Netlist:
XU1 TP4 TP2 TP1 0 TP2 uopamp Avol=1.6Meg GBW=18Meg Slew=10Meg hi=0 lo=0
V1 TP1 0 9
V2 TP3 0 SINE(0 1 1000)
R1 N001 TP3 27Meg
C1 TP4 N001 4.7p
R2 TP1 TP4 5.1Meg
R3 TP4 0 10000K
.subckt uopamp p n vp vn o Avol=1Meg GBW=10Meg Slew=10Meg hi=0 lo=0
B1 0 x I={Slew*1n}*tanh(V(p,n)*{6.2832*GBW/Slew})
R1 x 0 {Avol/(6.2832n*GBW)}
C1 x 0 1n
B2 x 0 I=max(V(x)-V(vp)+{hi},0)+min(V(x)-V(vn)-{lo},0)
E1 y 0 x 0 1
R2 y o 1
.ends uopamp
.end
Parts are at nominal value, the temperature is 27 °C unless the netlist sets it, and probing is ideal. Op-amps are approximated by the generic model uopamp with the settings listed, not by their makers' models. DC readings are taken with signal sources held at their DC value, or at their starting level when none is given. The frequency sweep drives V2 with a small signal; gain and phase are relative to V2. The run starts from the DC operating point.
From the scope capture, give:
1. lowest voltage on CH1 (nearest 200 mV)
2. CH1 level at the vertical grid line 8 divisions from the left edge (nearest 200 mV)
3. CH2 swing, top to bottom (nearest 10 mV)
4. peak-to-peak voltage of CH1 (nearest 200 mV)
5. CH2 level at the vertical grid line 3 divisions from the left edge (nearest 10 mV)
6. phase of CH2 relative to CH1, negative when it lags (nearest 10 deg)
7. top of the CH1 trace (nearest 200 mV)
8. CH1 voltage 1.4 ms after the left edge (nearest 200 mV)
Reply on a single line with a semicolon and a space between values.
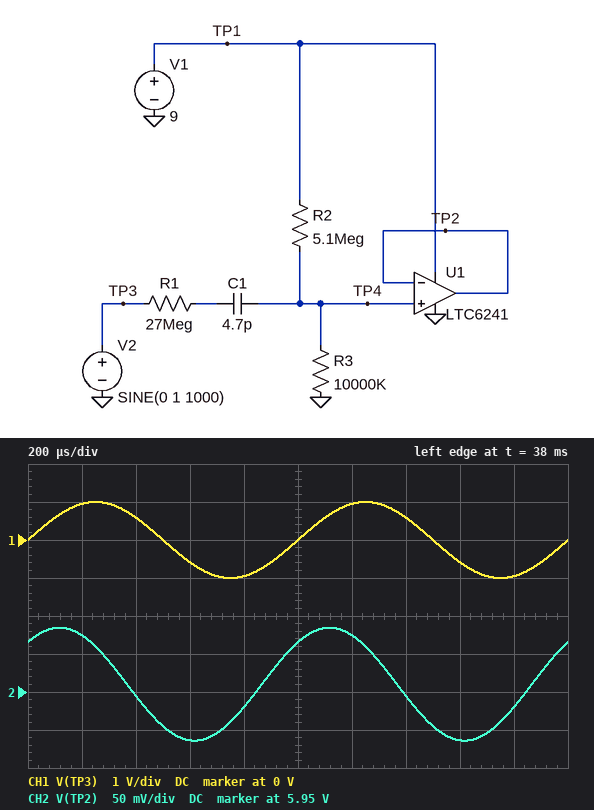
-1.0 V; -600 mV; 150 mV; 2.0 V; 5.89 V; 50 deg; 1.0 V; 600 mV
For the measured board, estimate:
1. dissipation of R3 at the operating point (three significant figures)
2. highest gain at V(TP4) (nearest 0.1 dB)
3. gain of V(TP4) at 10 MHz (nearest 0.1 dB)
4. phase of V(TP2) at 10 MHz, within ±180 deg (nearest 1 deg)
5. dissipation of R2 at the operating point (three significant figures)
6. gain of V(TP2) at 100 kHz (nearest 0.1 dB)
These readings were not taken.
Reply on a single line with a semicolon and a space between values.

3.55 µW; -19.1 dB; -19.1 dB; -29 deg; 1.81 µW; -19.1 dB
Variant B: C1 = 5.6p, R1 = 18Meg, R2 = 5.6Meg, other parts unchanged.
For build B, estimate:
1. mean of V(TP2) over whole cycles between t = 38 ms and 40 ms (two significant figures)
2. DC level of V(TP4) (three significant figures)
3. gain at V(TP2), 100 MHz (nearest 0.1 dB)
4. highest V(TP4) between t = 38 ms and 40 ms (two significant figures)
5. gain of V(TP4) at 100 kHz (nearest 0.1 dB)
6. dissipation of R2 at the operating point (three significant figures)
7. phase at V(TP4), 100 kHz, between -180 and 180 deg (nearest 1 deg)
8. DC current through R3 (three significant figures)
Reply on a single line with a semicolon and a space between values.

5.8 V; 5.77 V; -30.6 dB; 5.9 V; -15.6 dB; 1.86 µW; 1 deg; 577 nA
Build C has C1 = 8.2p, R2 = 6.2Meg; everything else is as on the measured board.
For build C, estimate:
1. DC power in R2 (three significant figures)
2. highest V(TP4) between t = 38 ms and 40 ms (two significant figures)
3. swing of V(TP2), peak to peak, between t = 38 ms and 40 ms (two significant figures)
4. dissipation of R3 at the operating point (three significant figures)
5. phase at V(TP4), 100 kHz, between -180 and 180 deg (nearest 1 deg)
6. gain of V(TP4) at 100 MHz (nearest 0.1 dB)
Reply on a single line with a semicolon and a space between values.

1.91 µW; 5.7 V; 210 mV; 3.09 µW; 0 deg; -18.1 dB
